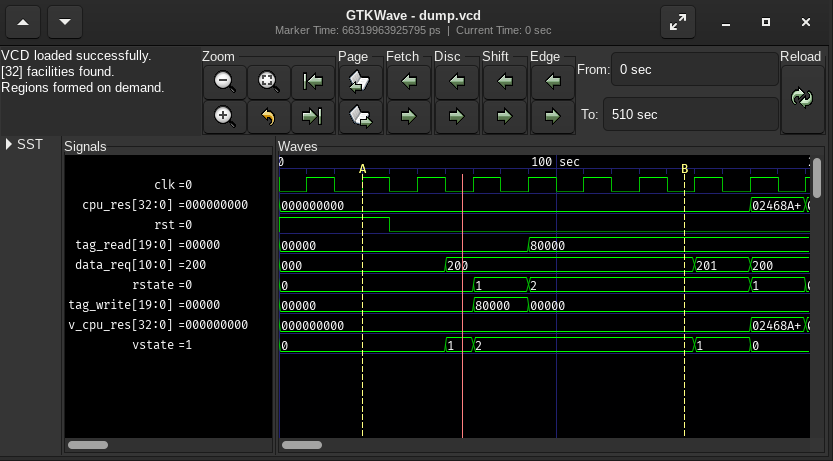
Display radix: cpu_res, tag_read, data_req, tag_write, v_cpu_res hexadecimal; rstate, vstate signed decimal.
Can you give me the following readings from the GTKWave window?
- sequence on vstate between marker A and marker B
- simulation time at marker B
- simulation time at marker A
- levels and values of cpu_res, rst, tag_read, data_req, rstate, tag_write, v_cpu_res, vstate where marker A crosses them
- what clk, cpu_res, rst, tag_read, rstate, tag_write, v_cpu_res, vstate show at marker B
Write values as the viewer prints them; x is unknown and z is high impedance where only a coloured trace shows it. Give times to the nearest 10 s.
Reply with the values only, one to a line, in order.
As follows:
0, 1, 2
150 s
30 s
cpu_res=000000000, rst=1, tag_read=00000, data_req=000, rstate=0, tag_write=00000, v_cpu_res=000000000, vstate=0
clk=0, cpu_res=000000000, rst=0, tag_read=80000, rstate=2, tag_write=00000, v_cpu_res=000000000, vstate=2
